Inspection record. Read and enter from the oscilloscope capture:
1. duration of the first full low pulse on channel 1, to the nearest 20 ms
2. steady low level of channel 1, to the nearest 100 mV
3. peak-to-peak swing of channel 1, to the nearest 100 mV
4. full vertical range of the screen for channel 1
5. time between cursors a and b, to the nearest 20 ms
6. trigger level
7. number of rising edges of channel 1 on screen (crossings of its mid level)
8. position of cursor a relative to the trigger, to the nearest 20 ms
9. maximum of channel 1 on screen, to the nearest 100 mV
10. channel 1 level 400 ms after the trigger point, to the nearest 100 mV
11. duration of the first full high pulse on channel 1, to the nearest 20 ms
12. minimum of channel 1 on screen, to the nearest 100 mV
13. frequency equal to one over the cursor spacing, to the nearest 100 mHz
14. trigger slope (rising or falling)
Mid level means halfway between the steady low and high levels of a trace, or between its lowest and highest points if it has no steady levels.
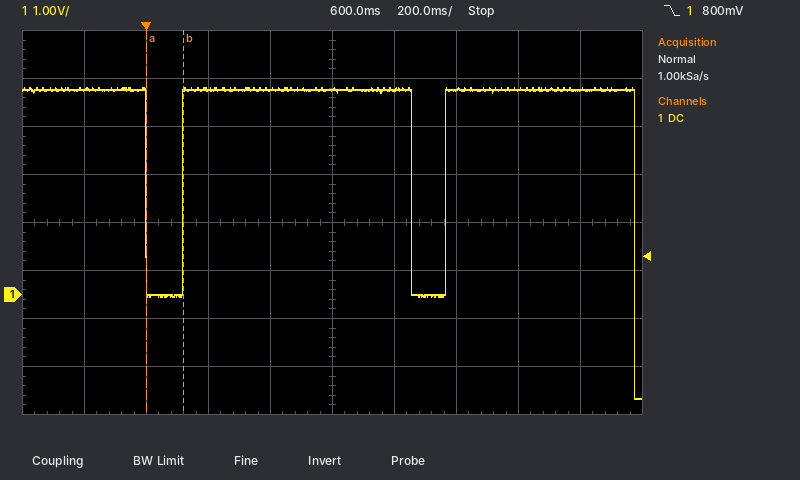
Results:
120 ms
0.0 V
6.5 V
8 V
120 ms
800 mV
2
0 ms
4.3 V
4.3 V
740 ms
-2.2 V
8.3 Hz
falling
